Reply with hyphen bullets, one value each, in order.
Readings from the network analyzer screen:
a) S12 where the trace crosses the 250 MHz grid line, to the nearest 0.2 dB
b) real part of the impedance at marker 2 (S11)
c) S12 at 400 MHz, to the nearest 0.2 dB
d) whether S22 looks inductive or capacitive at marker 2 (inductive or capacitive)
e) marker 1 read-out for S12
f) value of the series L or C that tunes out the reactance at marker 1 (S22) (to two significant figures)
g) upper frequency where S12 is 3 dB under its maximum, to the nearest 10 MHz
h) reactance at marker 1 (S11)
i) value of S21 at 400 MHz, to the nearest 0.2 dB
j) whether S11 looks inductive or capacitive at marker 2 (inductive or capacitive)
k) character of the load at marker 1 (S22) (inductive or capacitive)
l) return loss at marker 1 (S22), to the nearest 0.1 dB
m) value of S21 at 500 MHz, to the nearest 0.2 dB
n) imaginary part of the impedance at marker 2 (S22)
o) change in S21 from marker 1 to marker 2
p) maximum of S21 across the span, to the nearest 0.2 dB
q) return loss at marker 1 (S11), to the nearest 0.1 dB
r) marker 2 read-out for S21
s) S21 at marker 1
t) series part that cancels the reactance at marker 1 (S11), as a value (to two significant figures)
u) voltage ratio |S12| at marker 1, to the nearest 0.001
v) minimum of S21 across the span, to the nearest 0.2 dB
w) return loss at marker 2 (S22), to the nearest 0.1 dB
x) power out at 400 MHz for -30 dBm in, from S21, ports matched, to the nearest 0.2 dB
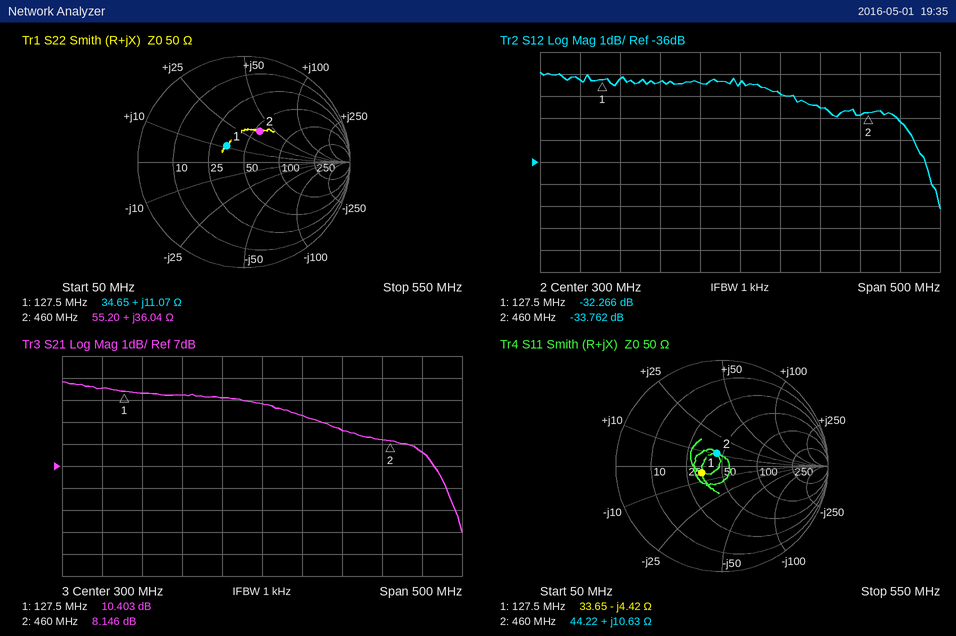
- -32.4 dB
- 44.22 Ω
- -33.6 dB
- inductive
- -32.266 dB
- 110 pF
- 520 MHz
- -4.42 Ω
- 8.6 dB
- inductive
- inductive
- 13.1 dB
- 7.6 dB
- +36.04 Ω
- -2.257 dB
- 10.8 dB
- 13.9 dB
- 8.146 dB
- 10.403 dB
- 5.5 nH
- 0.024
- 4.0 dB
- 9.7 dB
- -21.4 dBm
